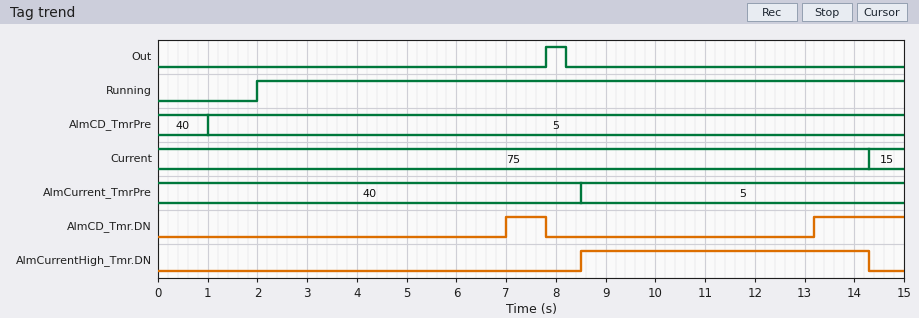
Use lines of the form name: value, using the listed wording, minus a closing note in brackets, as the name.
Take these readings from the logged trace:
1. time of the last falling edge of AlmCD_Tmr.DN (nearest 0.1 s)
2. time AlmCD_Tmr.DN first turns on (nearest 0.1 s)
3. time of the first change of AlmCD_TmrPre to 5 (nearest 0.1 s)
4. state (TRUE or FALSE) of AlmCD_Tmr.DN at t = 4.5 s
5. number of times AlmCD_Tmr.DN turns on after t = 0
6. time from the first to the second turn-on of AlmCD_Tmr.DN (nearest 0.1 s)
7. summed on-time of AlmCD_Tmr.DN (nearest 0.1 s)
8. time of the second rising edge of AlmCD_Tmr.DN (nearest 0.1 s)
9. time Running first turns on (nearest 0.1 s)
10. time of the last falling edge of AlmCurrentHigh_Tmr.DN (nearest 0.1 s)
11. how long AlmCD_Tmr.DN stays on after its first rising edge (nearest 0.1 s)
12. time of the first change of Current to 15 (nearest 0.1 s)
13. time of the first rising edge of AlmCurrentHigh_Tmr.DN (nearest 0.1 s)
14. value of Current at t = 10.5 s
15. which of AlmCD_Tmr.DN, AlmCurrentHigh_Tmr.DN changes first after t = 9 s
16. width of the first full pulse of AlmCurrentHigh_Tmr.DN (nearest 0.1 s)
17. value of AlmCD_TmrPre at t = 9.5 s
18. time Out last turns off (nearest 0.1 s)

time of the last falling edge of AlmCD_Tmr.DN: 7.8 s
time AlmCD_Tmr.DN first turns on: 7.0 s
time of the first change of AlmCD_TmrPre to 5: 1.0 s
state (TRUE or FALSE) of AlmCD_Tmr.DN at t = 4.5 s: FALSE
number of times AlmCD_Tmr.DN turns on after t = 0: 2
time from the first to the second turn-on of AlmCD_Tmr.DN: 6.2 s
summed on-time of AlmCD_Tmr.DN: 2.6 s
time of the second rising edge of AlmCD_Tmr.DN: 13.2 s
time Running first turns on: 2.0 s
time of the last falling edge of AlmCurrentHigh_Tmr.DN: 14.3 s
how long AlmCD_Tmr.DN stays on after its first rising edge: 0.8 s
time of the first change of Current to 15: 14.3 s
time of the first rising edge of AlmCurrentHigh_Tmr.DN: 8.5 s
value of Current at t = 10.5 s: 75
which of AlmCD_Tmr.DN, AlmCurrentHigh_Tmr.DN changes first after t = 9 s: AlmCD_Tmr.DN
width of the first full pulse of AlmCurrentHigh_Tmr.DN: 5.8 s
value of AlmCD_TmrPre at t = 9.5 s: 5
time Out last turns off: 8.2 s
